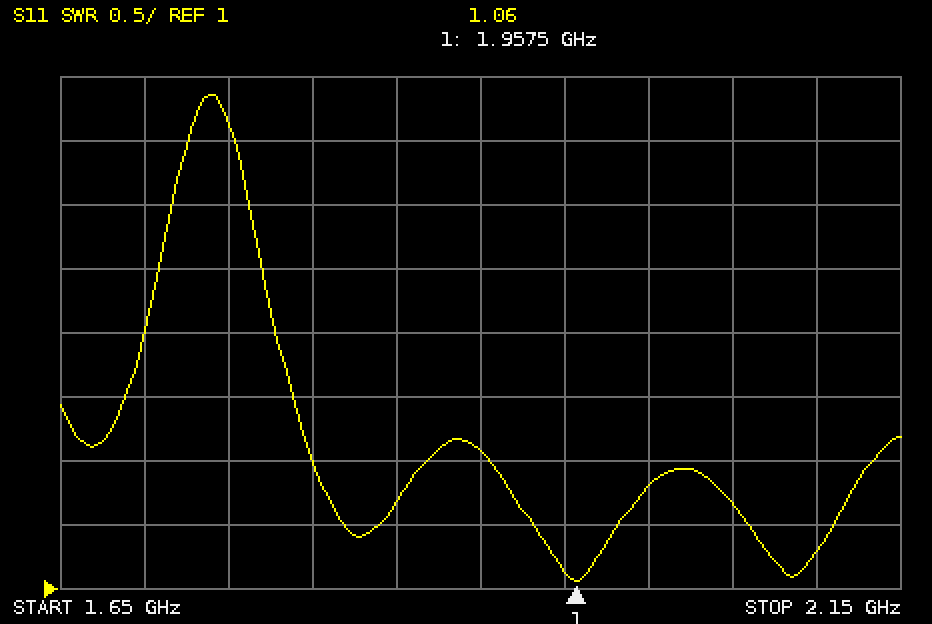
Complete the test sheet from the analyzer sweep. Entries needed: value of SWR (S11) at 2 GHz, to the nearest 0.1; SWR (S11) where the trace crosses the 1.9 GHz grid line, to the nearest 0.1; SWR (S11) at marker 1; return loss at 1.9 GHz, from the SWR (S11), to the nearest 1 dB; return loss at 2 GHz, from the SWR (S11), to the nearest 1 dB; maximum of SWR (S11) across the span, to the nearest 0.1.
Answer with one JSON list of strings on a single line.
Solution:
["1.8", "2.1", "1.06", "9 dB", "11 dB", "4.9"]
